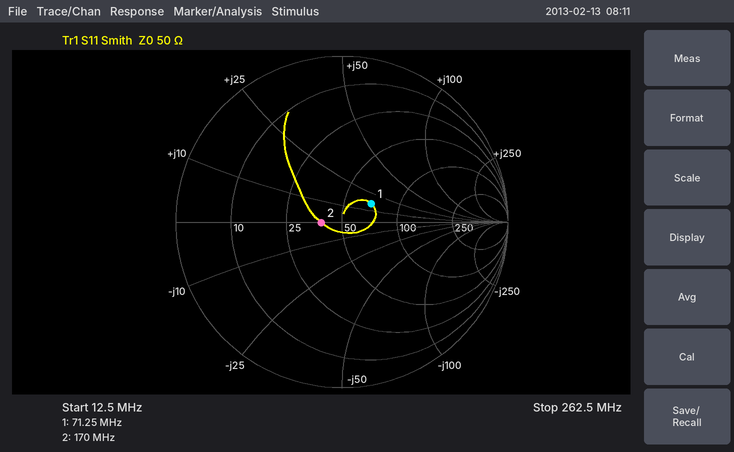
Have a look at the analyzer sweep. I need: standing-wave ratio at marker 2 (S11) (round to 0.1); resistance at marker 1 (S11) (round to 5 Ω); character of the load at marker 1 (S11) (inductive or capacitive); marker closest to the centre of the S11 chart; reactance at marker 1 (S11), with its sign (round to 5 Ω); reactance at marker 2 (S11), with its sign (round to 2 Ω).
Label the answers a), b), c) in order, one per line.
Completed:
a) 1.3
b) 70 Ω
c) inductive
d) marker 2
e) +15 Ω
f) 0 Ω
